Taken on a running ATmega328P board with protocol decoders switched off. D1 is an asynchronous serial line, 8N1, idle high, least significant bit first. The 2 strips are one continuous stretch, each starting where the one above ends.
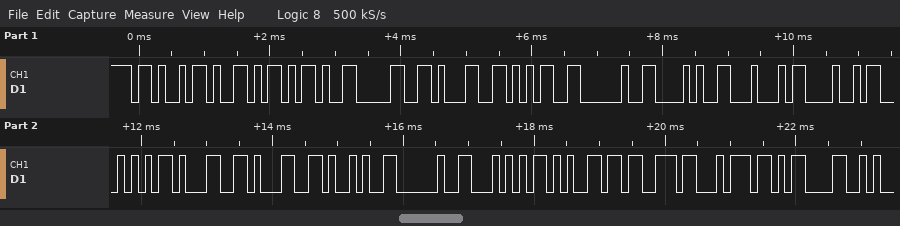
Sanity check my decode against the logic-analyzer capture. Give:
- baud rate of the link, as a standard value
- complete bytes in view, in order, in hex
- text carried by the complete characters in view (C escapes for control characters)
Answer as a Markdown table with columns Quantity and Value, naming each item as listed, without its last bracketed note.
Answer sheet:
| Quantity | Value |
|---|---|
| baud rate of the link, as a standard value | 9600 baud |
| complete bytes in view, in order, in hex | 4B 59 2D 30 31 35 20 28 44 48 54 31 31 29 20 54 65 73 74 0D |
| text carried by the complete characters in view | "KY-015 (DHT11) Test\r" |
